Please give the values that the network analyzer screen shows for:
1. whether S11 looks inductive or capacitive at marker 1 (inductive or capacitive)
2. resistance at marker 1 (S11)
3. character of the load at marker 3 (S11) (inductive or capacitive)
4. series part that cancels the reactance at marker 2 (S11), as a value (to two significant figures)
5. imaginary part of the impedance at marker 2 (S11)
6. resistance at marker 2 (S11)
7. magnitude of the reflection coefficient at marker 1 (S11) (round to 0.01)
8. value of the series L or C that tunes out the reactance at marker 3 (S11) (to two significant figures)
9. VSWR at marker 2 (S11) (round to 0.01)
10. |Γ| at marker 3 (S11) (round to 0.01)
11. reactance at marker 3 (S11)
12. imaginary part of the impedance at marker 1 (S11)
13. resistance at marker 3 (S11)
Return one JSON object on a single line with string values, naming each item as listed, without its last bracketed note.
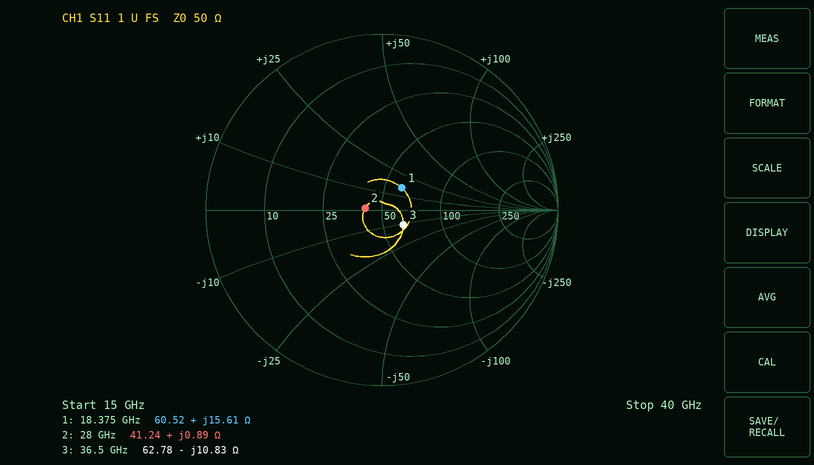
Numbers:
{"whether S11 looks inductive or capacitive at marker 1": "inductive", "resistance at marker 1": "60.52 Ω", "character of the load at marker 3 (S11)": "capacitive", "series part that cancels the reactance at marker 2 (S11), as a value": "6.4 pF", "imaginary part of the impedance at marker 2": "+0.89 Ω", "resistance at marker 2": "41.24 Ω", "magnitude of the reflection coefficient at marker 1 (S11)": "0.17", "value of the series L or C that tunes out the reactance at marker 3 (S11)": "47 pH", "VSWR at marker 2 (S11)": "1.21", "|Γ| at marker 3 (S11)": "0.15", "reactance at marker 3": "-10.83 Ω", "imaginary part of the impedance at marker 1": "+15.61 Ω", "resistance at marker 3": "62.78 Ω"}
